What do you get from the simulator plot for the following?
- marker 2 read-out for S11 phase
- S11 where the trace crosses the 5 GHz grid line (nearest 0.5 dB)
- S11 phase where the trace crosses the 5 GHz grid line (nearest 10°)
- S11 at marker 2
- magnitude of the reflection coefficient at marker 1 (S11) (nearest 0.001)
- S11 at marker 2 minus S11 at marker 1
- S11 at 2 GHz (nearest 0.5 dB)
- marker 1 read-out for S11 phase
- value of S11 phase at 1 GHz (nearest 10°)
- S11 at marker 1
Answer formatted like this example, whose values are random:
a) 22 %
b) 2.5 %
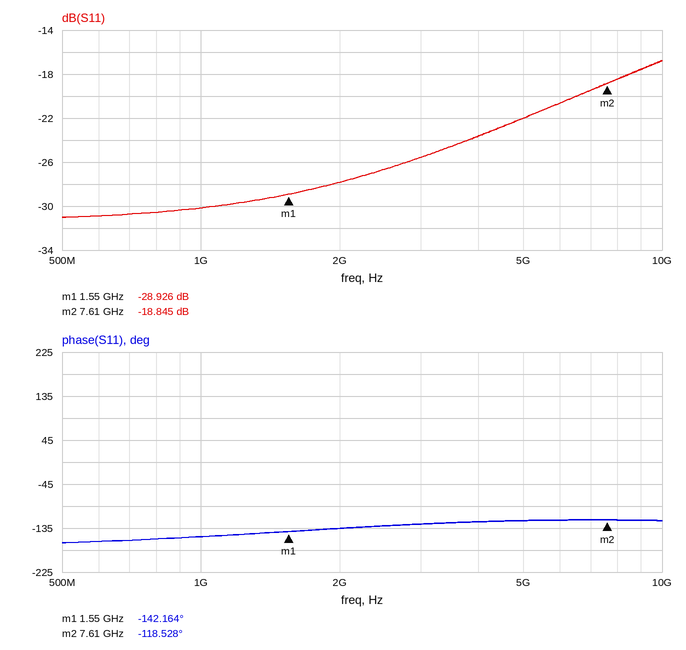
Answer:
a) -118.528°
b) -22.0 dB
c) -120°
d) -18.845 dB
e) 0.036
f) 10.081 dB
g) -28.0 dB
h) -142.164°
i) -150°
j) -28.926 dB
